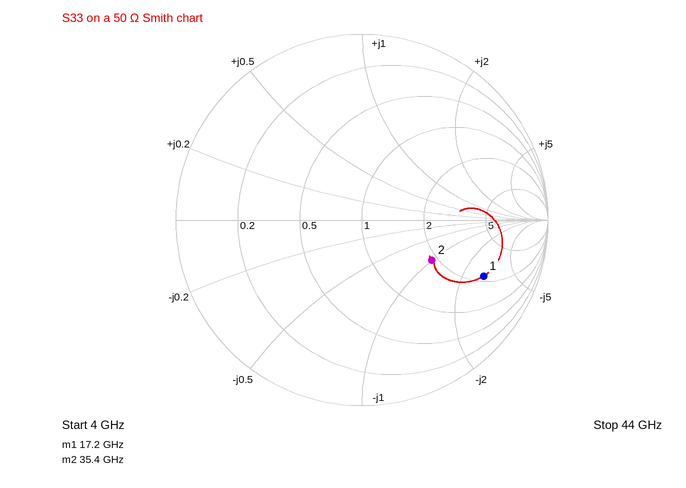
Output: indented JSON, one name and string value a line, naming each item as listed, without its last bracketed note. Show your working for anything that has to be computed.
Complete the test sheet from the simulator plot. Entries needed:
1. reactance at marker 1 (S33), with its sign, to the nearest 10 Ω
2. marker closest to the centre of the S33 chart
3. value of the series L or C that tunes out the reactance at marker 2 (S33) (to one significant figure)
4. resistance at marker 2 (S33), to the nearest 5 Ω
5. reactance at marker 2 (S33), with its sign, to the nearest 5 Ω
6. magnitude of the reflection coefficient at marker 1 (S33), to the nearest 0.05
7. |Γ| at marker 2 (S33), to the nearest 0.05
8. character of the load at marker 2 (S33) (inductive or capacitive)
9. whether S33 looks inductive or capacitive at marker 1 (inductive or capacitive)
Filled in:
{
  "reactance at marker 1 (S33), with its sign, to the nearest 10 Ω": "-140 Ω",
  "marker closest to the centre of the S33 chart": "marker 2",
  "value of the series L or C that tunes out the reactance at marker 2 (S33)": "L = 50 Ω/(2π × 35.4 GHz) ≈ 225 pH, so 200 pH to one significant figure",
  "resistance at marker 2 (S33), to the nearest 5 Ω": "95 Ω",
  "reactance at marker 2 (S33), with its sign, to the nearest 5 Ω": "-50 Ω",
  "magnitude of the reflection coefficient at marker 1 (S33), to the nearest 0.05": "0.70",
  "|Γ| at marker 2 (S33), to the nearest 0.05": "0.45",
  "character of the load at marker 2 (S33)": "capacitive",
  "whether S33 looks inductive or capacitive at marker 1": "capacitive"
}
